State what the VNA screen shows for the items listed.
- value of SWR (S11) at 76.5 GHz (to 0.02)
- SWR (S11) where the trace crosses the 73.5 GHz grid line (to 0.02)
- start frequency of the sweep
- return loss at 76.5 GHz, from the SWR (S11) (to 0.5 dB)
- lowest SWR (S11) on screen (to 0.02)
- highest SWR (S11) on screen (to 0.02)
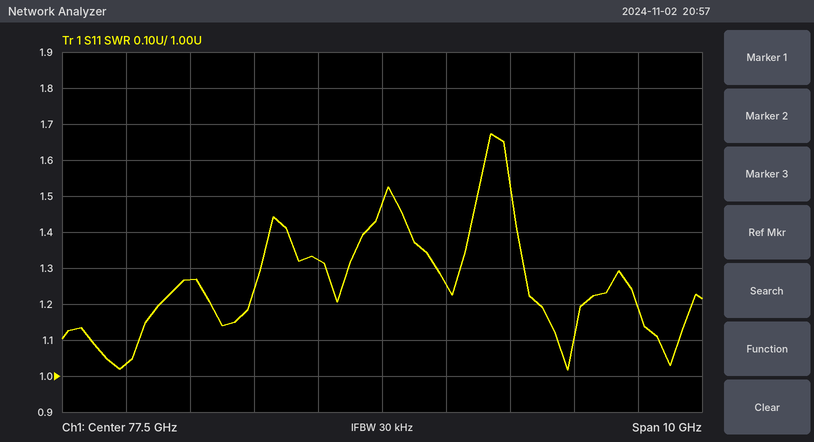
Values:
1.32
1.04
72.5 GHz
17.0 dB
1.02
1.68
